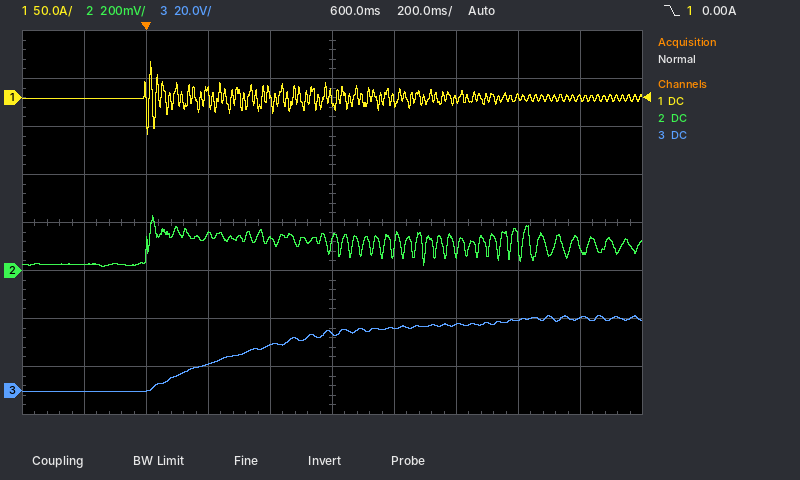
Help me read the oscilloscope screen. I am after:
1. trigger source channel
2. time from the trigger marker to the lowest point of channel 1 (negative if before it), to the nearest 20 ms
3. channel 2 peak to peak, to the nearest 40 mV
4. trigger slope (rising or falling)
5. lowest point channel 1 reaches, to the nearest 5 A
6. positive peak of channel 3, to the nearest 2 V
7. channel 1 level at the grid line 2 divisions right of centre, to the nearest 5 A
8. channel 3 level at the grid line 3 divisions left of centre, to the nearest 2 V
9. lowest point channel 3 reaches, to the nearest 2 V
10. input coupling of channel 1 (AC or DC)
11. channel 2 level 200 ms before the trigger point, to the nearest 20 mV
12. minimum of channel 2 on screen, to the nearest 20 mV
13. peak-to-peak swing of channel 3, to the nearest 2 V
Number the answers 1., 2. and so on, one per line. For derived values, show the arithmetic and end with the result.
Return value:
1. channel 1
2. 0 ms
3. 200 mV
4. falling
5. -40 A
6. 32 V
7. 0 A
8. 0 V
9. 0 V
10. DC
11. 20 mV
12. 20 mV
13. 32 V − (0 V) = 32 V
